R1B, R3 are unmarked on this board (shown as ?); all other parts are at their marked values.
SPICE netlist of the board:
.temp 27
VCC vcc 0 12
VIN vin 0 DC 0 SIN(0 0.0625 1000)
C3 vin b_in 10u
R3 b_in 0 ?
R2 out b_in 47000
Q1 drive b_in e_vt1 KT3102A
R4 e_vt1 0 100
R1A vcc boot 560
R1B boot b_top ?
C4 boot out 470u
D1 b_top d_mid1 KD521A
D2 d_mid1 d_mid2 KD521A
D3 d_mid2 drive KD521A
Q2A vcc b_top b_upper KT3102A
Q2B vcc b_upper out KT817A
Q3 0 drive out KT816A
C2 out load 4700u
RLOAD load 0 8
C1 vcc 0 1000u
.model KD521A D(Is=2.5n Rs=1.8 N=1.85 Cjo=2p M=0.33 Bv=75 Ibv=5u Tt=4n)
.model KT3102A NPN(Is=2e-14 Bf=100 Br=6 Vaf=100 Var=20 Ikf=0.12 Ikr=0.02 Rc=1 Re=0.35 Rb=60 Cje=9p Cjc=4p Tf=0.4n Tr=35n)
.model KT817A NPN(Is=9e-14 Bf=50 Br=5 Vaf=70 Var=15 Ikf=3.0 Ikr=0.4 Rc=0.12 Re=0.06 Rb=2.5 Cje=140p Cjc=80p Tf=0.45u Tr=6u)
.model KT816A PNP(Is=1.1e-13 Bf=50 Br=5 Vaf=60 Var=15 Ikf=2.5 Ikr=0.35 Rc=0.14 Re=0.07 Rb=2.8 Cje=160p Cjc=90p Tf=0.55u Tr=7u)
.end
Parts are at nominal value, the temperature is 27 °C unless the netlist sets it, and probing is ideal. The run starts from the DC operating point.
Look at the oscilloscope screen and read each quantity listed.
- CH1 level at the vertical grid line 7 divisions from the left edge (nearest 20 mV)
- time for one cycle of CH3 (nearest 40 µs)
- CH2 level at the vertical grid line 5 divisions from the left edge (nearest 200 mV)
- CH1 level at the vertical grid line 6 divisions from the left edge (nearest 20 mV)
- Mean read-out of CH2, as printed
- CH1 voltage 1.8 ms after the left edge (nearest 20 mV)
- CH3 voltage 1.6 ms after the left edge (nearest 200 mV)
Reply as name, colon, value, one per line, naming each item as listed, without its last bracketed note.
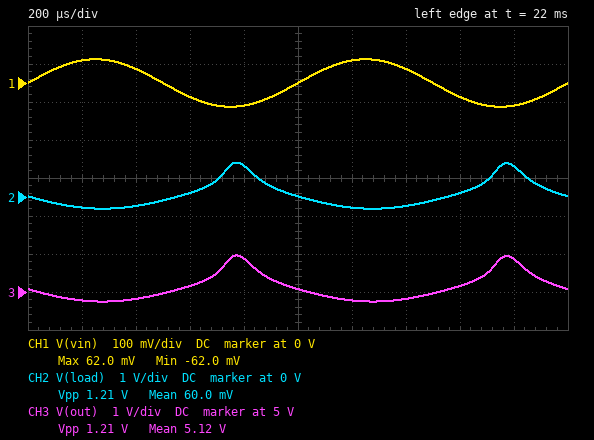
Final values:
CH1 level at the vertical grid line 7 divisions from the left edge: 40 mV
time for one cycle of CH3: 1.00 ms
CH2 level at the vertical grid line 5 divisions from the left edge: 0 V
CH1 level at the vertical grid line 6 divisions from the left edge: 60 mV
Mean read-out of CH2, as printed: 60.0 mV
CH1 voltage 1.8 ms after the left edge: -60 mV
CH3 voltage 1.6 ms after the left edge: 5.2 V
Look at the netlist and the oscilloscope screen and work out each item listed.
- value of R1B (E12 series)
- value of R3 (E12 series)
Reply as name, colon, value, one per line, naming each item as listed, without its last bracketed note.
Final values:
value of R1B: 2.2 kΩ
value of R3: 15 kΩ
